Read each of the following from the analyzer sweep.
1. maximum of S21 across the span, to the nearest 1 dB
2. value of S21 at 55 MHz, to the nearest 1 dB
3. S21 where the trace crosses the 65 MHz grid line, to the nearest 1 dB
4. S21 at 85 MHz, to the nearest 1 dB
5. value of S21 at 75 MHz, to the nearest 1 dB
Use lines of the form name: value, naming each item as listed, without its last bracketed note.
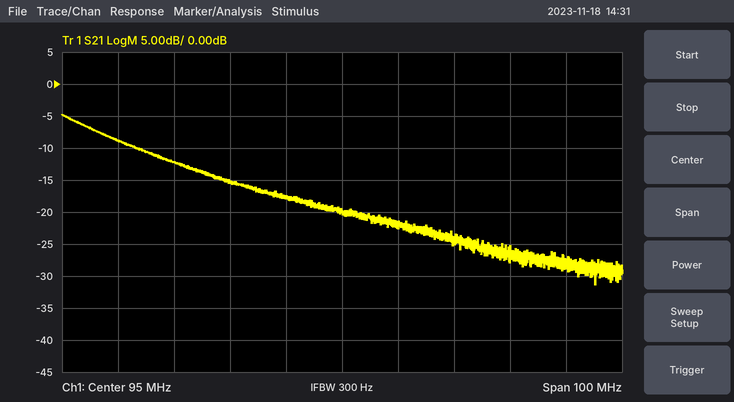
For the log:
maximum of S21 across the span, to the nearest 1 dB: -5 dB
value of S21 at 55 MHz, to the nearest 1 dB: -9 dB
S21 where the trace crosses the 65 MHz grid line, to the nearest 1 dB: -12 dB
S21 at 85 MHz, to the nearest 1 dB: -18 dB
value of S21 at 75 MHz, to the nearest 1 dB: -15 dB
